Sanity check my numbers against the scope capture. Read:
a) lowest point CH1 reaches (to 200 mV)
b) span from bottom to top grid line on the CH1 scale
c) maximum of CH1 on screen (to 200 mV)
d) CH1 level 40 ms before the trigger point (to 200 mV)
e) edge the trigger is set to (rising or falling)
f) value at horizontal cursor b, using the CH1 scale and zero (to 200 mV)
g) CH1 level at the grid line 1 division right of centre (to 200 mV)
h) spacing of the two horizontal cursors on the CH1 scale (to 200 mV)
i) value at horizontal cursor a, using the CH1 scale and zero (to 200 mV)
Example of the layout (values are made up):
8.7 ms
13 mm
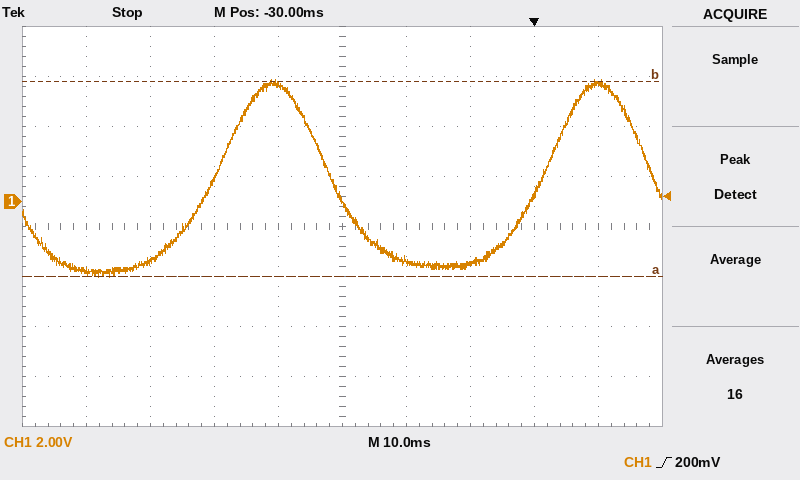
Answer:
-3.0 V
16 V
4.8 V
4.6 V
rising
4.8 V
-2.4 V
7.8 V
-3.0 V
